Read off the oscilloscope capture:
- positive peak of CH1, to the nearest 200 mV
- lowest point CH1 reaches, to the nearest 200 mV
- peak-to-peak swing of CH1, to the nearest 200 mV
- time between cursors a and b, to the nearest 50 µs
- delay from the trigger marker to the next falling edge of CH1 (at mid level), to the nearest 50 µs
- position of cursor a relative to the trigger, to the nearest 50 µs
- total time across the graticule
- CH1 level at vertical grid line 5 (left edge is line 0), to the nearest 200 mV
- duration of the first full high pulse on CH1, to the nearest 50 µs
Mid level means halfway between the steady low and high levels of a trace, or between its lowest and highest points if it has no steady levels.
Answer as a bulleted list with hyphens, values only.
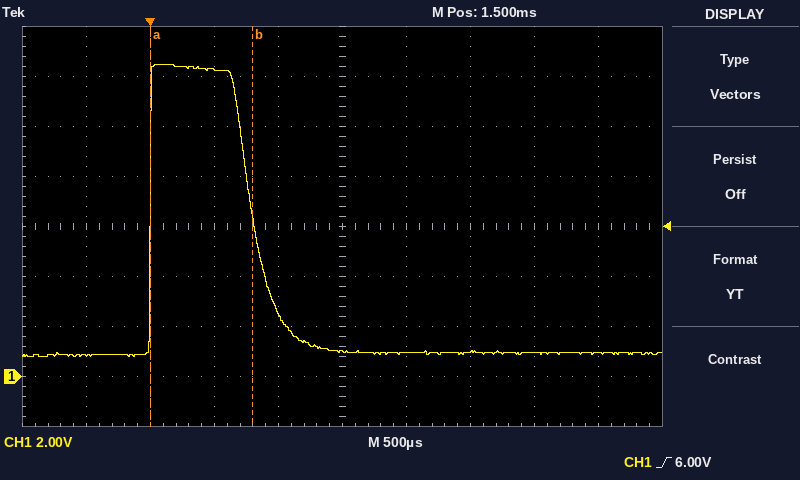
- 12.4 V
- 800 mV
- 11.6 V
- 800 µs
- 800 µs
- 0 µs
- 5 ms
- 1.0 V
- 800 µs
